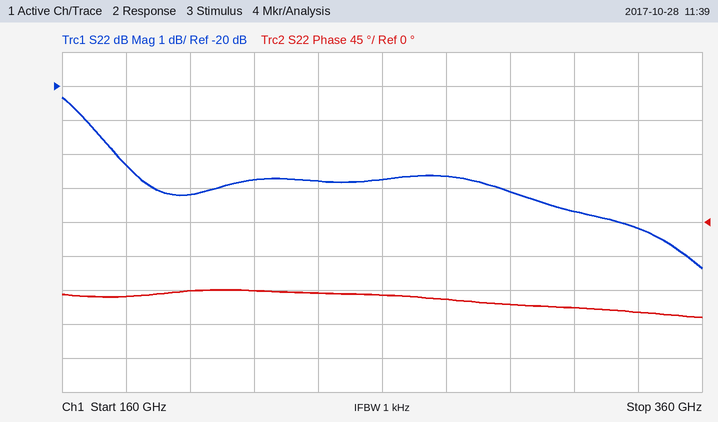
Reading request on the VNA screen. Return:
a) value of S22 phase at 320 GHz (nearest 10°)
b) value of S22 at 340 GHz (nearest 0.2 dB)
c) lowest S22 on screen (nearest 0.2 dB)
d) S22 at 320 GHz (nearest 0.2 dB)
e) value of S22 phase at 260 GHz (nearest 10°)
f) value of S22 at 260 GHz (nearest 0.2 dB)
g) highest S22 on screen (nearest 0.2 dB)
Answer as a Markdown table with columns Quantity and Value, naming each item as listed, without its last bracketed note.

| Quantity | Value |
|---|---|
| value of S22 phase at 320 GHz | -110° |
| value of S22 at 340 GHz | -24.2 dB |
| lowest S22 on screen | -25.4 dB |
| S22 at 320 GHz | -23.6 dB |
| value of S22 phase at 260 GHz | -100° |
| value of S22 at 260 GHz | -22.8 dB |
| highest S22 on screen | -20.4 dB |
